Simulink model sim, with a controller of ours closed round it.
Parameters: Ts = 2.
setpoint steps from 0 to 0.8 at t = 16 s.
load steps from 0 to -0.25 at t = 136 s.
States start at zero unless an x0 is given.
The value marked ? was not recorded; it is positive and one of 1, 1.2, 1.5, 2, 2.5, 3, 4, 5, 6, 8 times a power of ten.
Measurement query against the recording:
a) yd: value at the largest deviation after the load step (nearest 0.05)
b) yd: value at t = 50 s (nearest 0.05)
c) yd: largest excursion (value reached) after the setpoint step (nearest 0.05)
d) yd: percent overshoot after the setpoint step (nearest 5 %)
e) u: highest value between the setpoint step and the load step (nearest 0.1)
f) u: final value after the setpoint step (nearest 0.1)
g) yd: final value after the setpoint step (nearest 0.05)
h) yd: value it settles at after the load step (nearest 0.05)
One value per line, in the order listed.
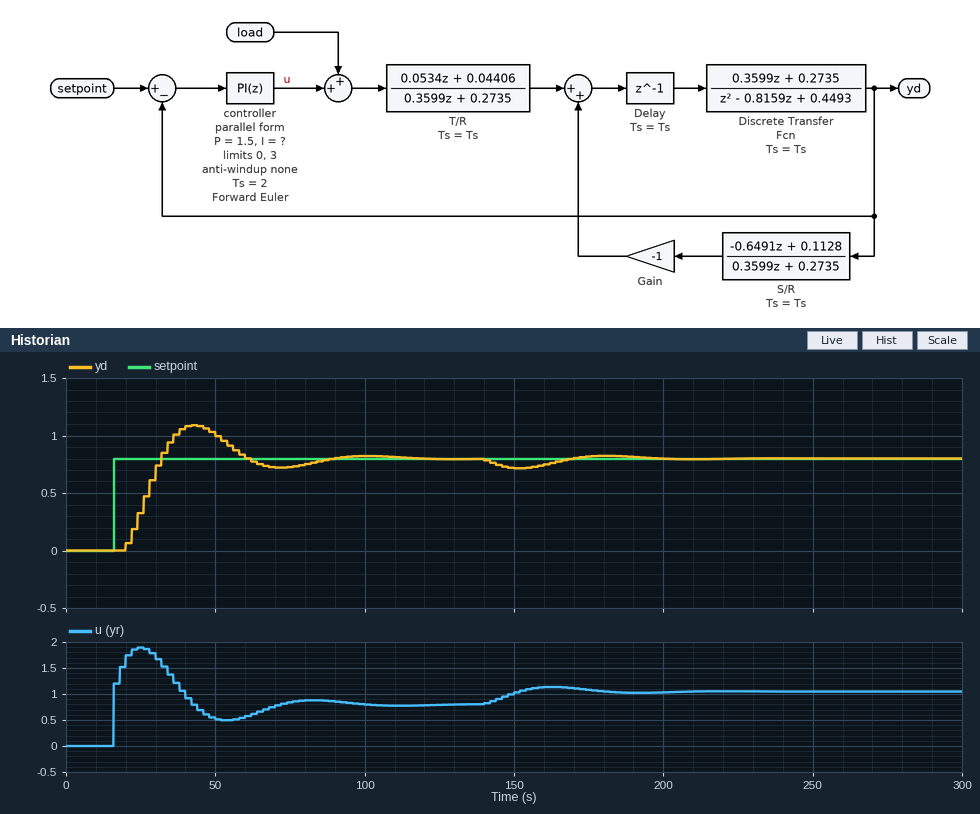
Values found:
0.70
1.00
1.10
35 %
1.9
0.8
0.80
0.80
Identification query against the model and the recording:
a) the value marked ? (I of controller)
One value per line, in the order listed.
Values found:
0.2
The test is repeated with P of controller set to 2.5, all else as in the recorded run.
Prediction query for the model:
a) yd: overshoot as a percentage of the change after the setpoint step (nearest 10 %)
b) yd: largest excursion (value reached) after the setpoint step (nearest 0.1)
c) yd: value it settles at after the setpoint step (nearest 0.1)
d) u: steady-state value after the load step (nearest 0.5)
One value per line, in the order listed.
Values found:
20 %
1.0
0.8
1.0
